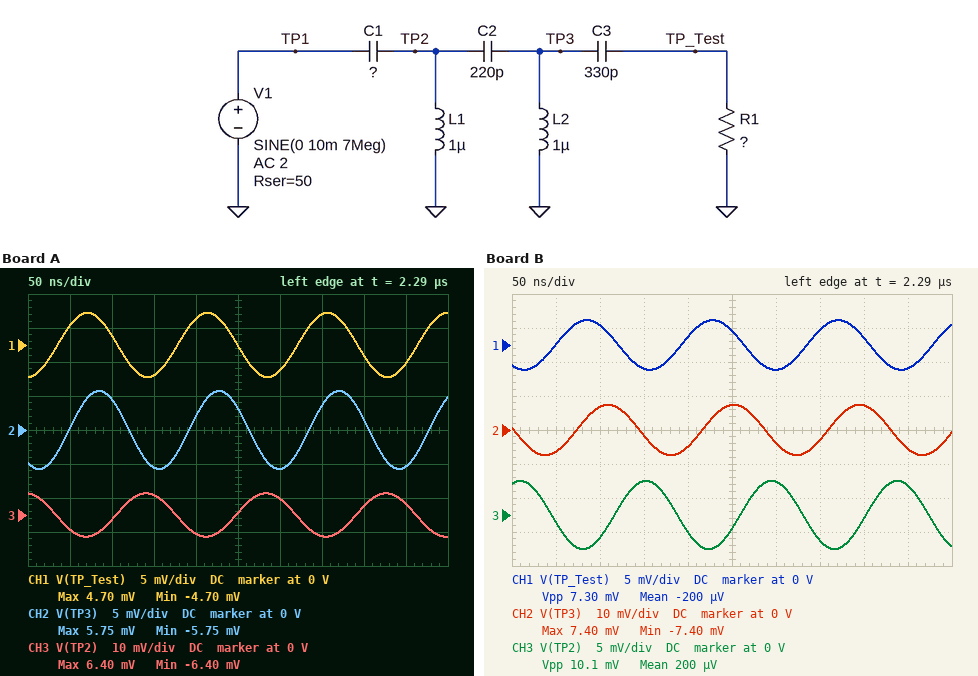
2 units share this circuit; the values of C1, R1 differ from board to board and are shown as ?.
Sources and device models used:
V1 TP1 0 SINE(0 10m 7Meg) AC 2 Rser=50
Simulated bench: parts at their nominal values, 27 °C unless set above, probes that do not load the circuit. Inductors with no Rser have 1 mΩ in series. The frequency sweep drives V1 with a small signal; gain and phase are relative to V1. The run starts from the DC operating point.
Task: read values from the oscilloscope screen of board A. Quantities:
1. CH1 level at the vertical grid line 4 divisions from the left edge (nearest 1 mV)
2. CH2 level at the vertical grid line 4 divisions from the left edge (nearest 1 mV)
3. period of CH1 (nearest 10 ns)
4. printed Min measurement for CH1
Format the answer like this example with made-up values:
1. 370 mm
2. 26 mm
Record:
1. 4 mV
2. 2 mV
3. 140 ns
4. -4.70 mV
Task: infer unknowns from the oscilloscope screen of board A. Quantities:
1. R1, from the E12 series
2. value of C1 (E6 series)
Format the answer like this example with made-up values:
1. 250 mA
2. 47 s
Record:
1. 100 Ω
2. 100 pF
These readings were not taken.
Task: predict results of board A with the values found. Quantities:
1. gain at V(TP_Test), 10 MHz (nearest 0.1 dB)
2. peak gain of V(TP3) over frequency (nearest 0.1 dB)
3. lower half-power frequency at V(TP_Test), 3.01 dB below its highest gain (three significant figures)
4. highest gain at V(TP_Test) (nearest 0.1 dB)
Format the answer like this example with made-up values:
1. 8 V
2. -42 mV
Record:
1. -8.6 dB
2. -3.0 dB
3. 13.6 MHz
4. -3.2 dB
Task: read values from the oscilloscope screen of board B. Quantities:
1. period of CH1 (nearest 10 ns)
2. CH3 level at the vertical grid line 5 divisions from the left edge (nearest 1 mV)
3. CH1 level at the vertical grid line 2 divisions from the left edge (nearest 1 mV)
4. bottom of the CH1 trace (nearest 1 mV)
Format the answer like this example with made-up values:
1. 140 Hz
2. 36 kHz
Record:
1. 140 ns
2. -2 mV
3. 3 mV
4. -4 mV
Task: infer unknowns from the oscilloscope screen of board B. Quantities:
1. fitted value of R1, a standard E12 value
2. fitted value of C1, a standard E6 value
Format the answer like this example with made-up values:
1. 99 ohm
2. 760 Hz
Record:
1. 39 Ω
2. 220 pF
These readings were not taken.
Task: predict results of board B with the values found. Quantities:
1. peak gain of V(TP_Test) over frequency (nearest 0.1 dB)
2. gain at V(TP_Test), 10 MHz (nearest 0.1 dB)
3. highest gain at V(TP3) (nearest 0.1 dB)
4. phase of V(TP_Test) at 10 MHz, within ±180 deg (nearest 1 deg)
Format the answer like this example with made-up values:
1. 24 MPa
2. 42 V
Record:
1. -7.1 dB
2. -7.3 dB
3. -0.9 dB
4. 158 deg
